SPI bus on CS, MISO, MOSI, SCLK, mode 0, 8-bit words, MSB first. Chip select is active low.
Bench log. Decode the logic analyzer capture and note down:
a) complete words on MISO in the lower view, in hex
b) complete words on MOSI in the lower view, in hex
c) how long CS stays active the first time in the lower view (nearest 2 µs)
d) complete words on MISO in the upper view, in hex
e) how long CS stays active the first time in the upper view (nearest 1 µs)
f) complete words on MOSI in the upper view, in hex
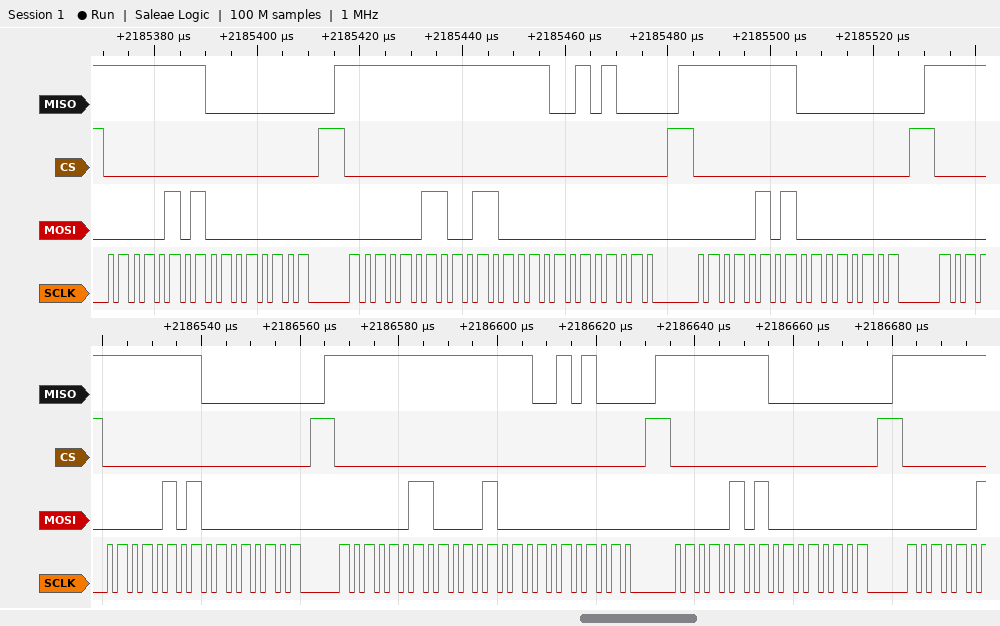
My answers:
FF, 00, FF, FF, 28, FF, 00
05, 00, 03, 08, 00, 05, 00
42 µs
FF, 00, FF, FF, 28, FF, 00
42 µs
05, 00, 03, 30, 00, 05, 00
